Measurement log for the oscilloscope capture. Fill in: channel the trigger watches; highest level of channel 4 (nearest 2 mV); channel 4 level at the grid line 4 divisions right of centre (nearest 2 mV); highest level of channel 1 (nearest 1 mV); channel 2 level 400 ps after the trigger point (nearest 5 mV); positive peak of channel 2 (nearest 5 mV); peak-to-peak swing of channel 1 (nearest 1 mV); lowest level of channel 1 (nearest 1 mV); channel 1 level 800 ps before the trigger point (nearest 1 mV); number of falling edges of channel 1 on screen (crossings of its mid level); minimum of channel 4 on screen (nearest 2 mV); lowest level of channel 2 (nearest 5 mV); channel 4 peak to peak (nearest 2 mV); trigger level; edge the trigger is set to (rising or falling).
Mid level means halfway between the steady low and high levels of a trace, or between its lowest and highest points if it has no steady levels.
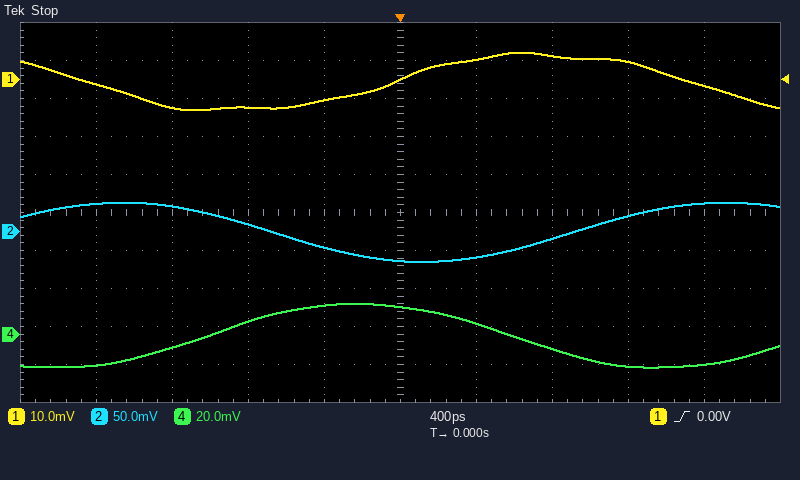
channel 1
16 mV
-16 mV
7 mV
-35 mV
40 mV
15 mV
-8 mV
-7 mV
2
-18 mV
-40 mV
34 mV
0.00 V
rising
